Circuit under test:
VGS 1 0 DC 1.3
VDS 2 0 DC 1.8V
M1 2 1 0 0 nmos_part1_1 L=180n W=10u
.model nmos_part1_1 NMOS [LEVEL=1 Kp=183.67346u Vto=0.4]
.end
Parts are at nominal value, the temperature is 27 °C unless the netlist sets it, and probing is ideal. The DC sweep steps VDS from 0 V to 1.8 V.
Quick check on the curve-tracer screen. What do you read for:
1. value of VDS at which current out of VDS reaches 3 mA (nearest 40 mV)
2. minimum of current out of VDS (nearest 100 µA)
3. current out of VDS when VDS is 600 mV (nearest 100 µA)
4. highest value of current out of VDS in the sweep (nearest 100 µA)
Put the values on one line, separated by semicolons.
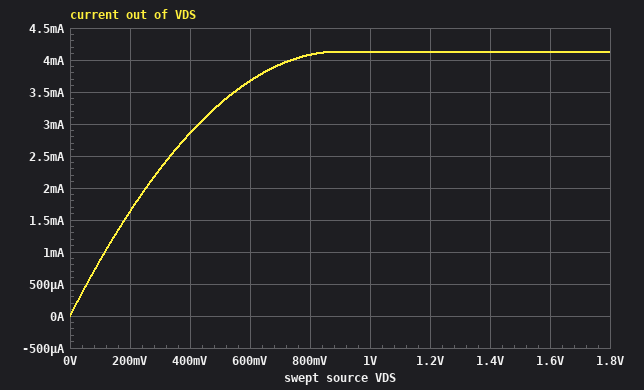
440 mV; 0 A; 3.7 mA; 4.1 mA
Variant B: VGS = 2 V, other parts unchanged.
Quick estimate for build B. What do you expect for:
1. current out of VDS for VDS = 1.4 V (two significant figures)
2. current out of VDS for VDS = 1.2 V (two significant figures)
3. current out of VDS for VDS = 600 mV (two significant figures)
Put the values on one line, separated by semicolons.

13 mA; 12 mA; 8.0 mA
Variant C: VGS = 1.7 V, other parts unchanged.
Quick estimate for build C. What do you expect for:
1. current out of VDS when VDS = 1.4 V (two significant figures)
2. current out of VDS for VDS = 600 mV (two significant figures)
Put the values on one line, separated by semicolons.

8.6 mA; 6.1 mA
